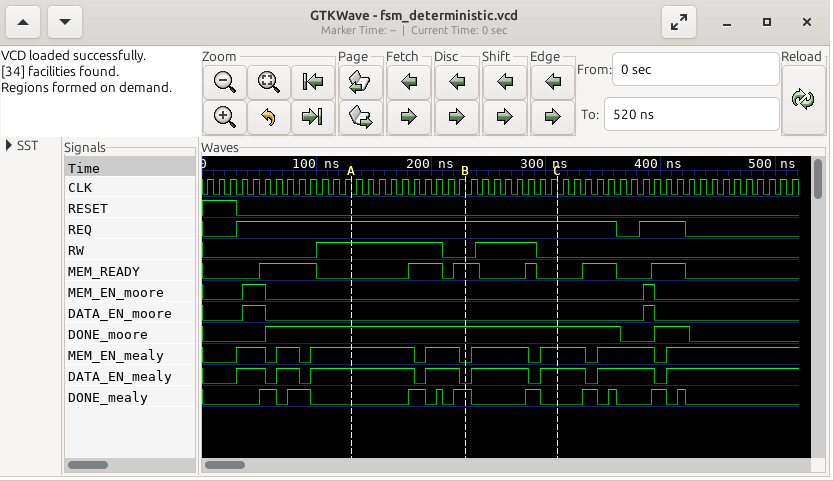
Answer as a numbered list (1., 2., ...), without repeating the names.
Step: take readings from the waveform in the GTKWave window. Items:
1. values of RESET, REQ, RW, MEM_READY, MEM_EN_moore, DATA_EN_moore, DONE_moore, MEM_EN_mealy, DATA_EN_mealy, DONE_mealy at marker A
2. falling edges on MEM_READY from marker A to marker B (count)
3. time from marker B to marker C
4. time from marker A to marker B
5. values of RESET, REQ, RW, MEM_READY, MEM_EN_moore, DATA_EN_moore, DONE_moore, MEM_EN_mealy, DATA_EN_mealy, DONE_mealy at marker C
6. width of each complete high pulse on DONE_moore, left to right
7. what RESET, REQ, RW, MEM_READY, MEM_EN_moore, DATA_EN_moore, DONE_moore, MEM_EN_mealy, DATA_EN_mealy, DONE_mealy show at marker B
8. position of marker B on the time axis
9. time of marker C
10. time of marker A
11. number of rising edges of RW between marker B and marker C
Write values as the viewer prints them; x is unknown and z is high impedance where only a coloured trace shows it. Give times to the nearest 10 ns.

1. RESET=0, REQ=1, RW=1, MEM_READY=0, MEM_EN_moore=0, DATA_EN_moore=0, DONE_moore=1, MEM_EN_mealy=1, DATA_EN_mealy=1, DONE_mealy=0
2. 1
3. 80 ns
4. 100 ns
5. RESET=0, REQ=1, RW=0, MEM_READY=0, MEM_EN_moore=0, DATA_EN_moore=0, DONE_moore=1, MEM_EN_mealy=1, DATA_EN_mealy=1, DONE_mealy=0
6. 310 ns, 30 ns
7. RESET=0, REQ=1, RW=0, MEM_READY=1, MEM_EN_moore=0, DATA_EN_moore=0, DONE_moore=1, MEM_EN_mealy=0, DATA_EN_mealy=0, DONE_mealy=1
8. 230 ns
9. 310 ns
10. 130 ns
11. 1
